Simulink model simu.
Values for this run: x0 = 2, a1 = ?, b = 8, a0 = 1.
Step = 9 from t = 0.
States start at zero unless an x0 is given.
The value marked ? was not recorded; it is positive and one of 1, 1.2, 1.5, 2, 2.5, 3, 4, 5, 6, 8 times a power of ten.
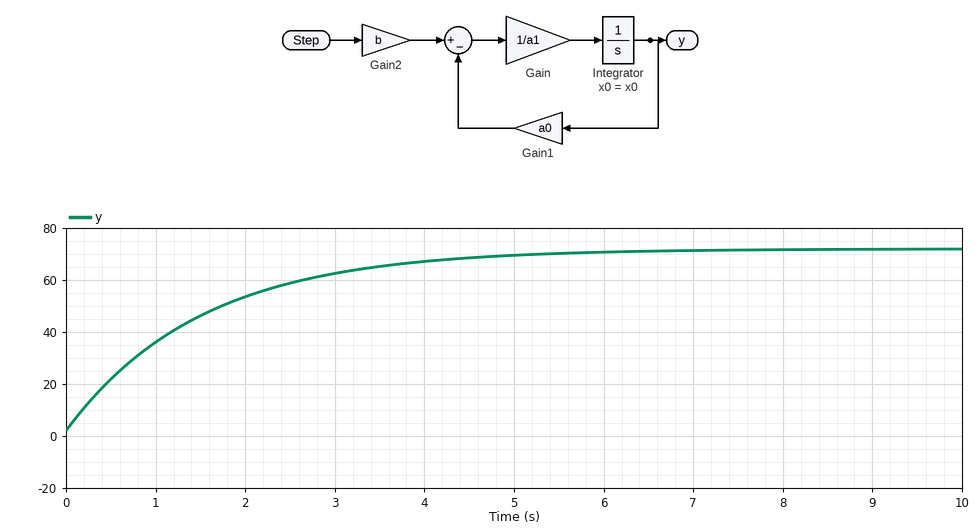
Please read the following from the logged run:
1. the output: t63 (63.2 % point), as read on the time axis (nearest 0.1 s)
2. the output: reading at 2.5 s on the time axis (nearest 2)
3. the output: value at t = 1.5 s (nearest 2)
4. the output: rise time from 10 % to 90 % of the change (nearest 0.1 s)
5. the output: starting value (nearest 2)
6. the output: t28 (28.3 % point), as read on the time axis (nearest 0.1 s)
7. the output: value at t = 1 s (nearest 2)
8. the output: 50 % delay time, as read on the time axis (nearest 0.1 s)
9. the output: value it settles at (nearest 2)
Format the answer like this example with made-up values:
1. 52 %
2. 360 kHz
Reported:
1. 1.5 s
2. 58
3. 46
4. 3.3 s
5. 2
6. 0.5 s
7. 36
8. 1.0 s
9. 72
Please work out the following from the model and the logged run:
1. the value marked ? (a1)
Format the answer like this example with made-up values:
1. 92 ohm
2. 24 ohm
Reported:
1. 1.5
